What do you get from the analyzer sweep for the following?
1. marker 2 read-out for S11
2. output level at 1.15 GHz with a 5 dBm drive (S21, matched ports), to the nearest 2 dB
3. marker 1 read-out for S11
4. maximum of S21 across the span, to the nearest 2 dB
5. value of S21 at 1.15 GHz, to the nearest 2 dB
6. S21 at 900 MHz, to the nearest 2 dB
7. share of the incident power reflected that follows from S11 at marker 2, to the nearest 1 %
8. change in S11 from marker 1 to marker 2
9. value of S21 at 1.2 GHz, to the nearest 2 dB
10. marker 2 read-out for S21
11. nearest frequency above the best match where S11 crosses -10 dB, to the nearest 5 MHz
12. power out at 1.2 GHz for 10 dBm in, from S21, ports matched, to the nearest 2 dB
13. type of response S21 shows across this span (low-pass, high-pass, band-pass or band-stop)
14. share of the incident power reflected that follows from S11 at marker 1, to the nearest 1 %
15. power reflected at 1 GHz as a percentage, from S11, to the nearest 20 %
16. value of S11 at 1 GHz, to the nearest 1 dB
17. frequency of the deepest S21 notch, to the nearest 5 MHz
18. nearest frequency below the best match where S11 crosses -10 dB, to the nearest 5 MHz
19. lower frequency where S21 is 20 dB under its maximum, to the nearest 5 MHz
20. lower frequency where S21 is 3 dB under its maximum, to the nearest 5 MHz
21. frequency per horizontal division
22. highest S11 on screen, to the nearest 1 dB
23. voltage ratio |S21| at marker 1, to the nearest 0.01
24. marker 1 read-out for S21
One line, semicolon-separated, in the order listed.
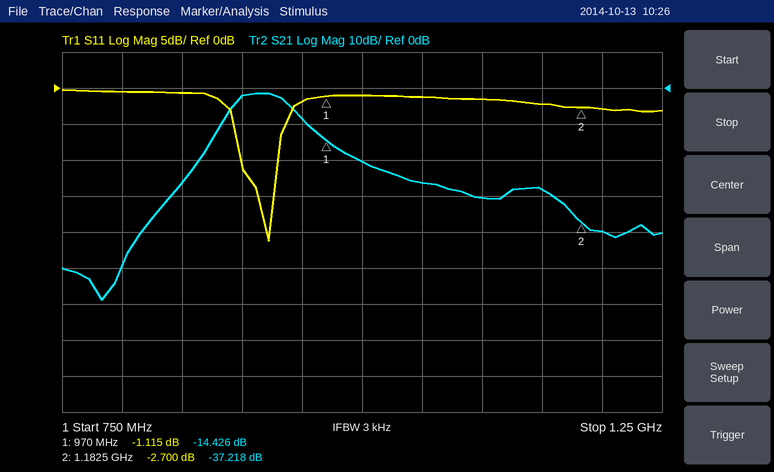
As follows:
-2.700 dB; -24 dBm; -1.115 dB; -2 dB; -28 dB; -2 dB; 54 %; -1.585 dB; -40 dB; -37.218 dB; 930 MHz; -30 dBm; band-pass; 77 %; 80 %; -1 dB; 785 MHz; 900 MHz; 860 MHz; 895 MHz; 50 MHz; 0 dB; 0.19; -14.426 dB
